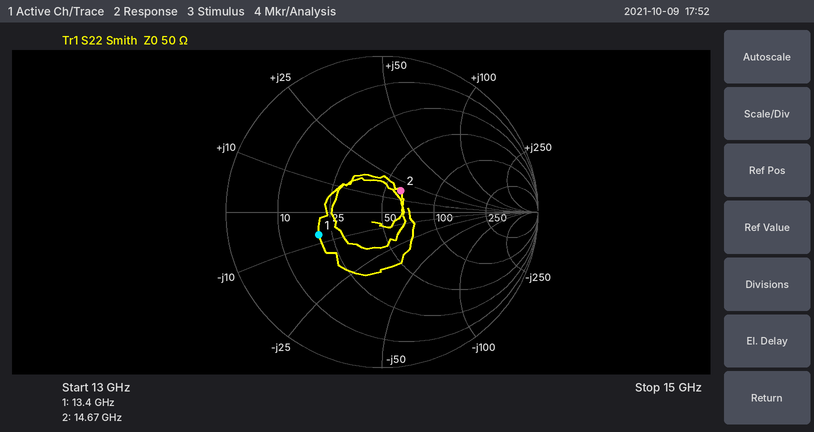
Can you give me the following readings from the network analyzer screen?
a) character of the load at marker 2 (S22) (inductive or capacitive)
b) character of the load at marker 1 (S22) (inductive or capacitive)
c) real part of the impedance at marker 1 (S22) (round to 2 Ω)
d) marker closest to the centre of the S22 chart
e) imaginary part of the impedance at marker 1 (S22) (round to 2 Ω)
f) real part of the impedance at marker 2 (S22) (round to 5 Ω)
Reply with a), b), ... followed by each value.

a) inductive
b) capacitive
c) 20 Ω
d) marker 2
e) -8 Ω
f) 60 Ω
